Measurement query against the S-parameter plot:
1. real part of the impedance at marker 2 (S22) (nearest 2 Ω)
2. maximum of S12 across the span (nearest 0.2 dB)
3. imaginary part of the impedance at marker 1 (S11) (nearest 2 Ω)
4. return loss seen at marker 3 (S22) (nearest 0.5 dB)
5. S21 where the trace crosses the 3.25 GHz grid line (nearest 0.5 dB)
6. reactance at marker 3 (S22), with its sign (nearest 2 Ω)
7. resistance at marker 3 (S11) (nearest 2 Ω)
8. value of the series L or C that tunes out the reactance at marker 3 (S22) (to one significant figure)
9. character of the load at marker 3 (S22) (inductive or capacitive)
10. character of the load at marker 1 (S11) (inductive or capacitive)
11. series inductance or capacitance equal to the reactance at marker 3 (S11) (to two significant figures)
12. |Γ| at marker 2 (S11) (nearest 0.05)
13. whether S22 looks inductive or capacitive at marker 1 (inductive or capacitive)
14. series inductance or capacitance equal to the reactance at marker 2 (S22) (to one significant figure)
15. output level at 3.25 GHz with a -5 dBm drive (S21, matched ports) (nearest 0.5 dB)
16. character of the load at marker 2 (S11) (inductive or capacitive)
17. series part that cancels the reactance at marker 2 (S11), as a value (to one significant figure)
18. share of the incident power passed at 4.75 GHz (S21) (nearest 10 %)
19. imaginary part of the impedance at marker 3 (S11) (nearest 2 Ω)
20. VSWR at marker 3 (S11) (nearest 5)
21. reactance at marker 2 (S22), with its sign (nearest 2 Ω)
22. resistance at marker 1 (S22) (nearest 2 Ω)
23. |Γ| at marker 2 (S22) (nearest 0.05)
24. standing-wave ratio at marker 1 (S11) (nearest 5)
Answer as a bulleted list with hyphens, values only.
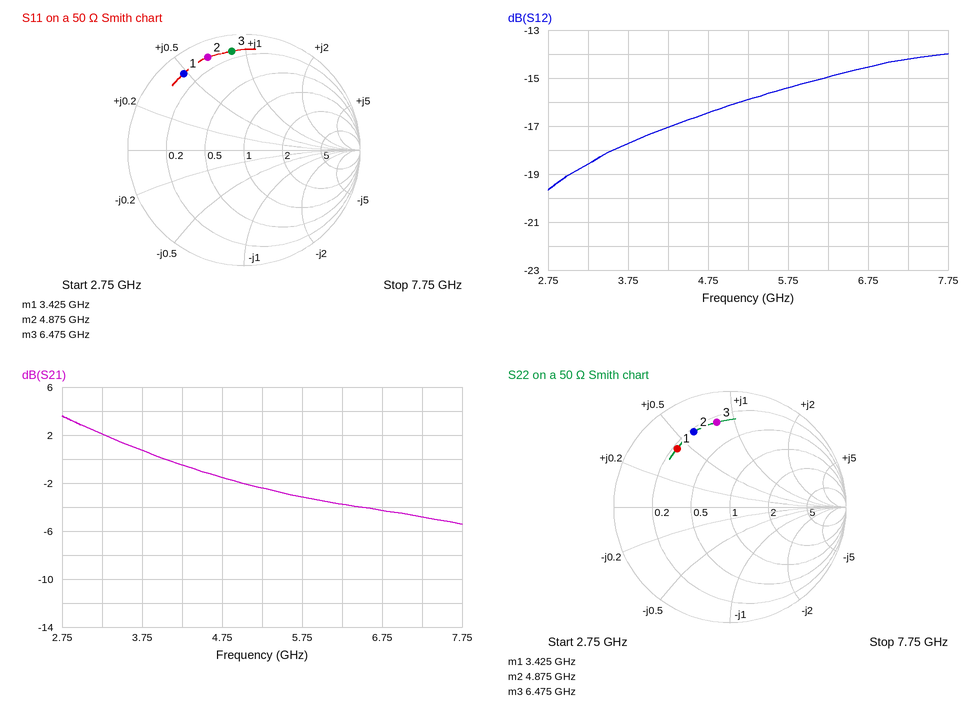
- 12 Ω
- -14.0 dB
- +24 Ω
- 2.5 dB
- 2.0 dB
- +42 Ω
- 6 Ω
- 600 fF
- inductive
- inductive
- 1.1 nH
- 0.85
- inductive
- 1.0 nH
- -3.0 dBm
- inductive
- 1.0 pF
- 70 %
- +44 Ω
- 15
- +30 Ω
- 12 Ω
- 0.70
- 10
